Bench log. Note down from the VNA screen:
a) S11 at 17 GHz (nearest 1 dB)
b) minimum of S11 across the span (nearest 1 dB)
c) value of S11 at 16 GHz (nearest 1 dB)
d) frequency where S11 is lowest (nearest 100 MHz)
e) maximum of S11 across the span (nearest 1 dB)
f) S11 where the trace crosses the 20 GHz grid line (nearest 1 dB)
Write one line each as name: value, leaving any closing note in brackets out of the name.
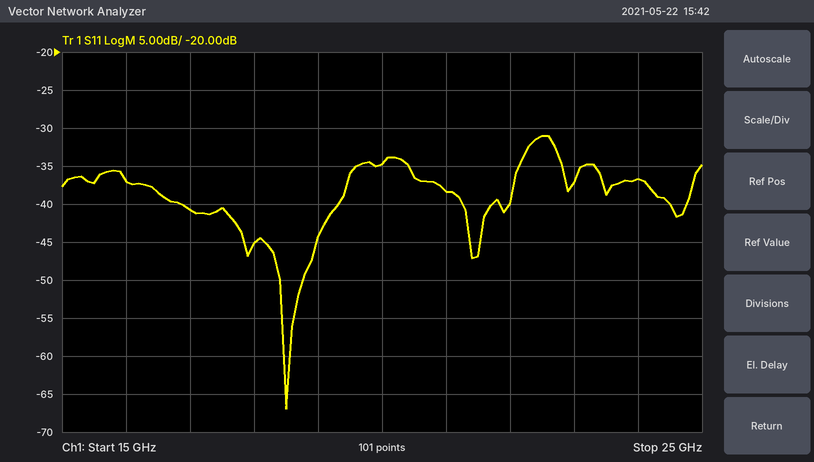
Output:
S11 at 17 GHz: -41 dB
minimum of S11 across the span: -67 dB
value of S11 at 16 GHz: -37 dB
frequency where S11 is lowest: 18.5 GHz
maximum of S11 across the span: -31 dB
S11 where the trace crosses the 20 GHz grid line: -35 dB
